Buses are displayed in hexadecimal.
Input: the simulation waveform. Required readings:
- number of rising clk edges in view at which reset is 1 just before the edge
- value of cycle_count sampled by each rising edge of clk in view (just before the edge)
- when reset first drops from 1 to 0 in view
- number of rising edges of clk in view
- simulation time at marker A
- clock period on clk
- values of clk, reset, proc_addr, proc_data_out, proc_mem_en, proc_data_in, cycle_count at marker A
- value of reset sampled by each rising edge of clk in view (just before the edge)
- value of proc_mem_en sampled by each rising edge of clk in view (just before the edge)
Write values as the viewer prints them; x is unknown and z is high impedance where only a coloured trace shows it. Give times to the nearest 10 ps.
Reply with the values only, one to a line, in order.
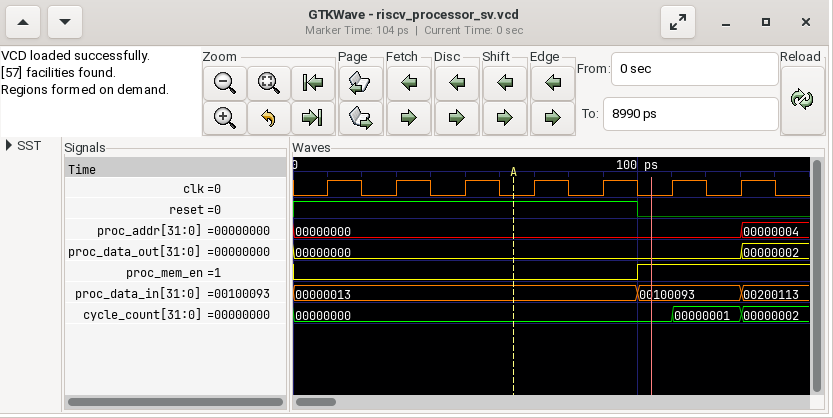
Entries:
5
00000000, 00000000, 00000000, 00000000, 00000000, 00000000, 00000001
100 ps
7
60 ps
20 ps
clk=0, reset=1, proc_addr=00000000, proc_data_out=00000000, proc_mem_en=0, proc_data_in=00000013, cycle_count=00000000
1 1 1 1 1 0 0
0 0 0 0 0 1 1
